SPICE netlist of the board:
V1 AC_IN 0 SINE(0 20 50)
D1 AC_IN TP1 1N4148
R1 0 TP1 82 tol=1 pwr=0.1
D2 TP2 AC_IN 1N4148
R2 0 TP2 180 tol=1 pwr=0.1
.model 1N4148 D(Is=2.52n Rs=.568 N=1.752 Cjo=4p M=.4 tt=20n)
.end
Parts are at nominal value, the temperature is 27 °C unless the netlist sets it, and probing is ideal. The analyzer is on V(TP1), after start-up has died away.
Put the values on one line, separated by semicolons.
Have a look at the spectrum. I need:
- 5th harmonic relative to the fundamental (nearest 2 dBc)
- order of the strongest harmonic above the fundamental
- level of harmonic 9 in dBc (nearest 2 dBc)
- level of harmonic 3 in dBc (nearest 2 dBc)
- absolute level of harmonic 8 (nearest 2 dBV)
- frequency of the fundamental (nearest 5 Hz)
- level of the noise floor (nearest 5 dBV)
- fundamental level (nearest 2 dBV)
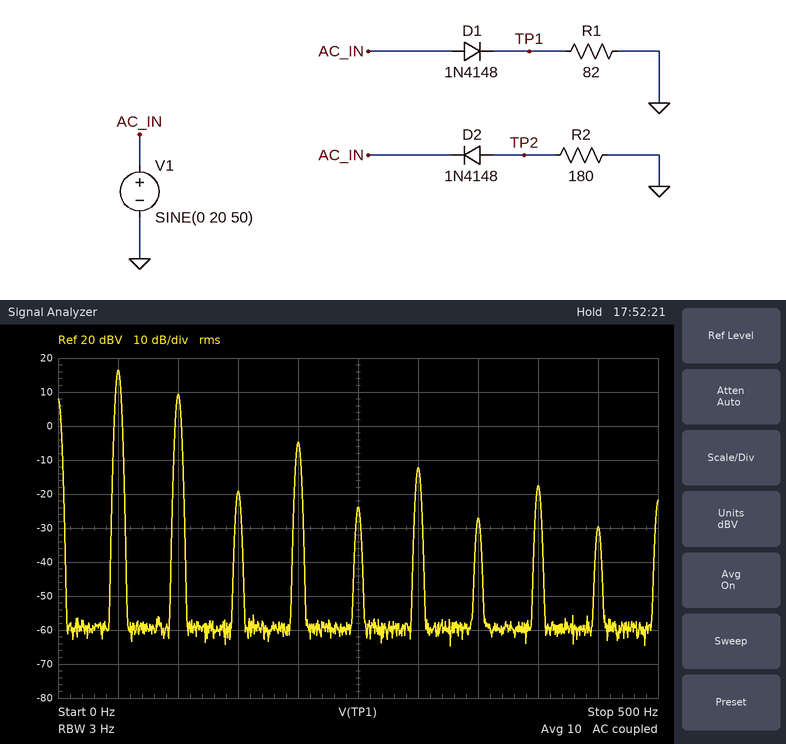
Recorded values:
-40 dBc; 2; -46 dBc; -36 dBc; -18 dBV; 50 Hz; -60 dBV; 16 dBV
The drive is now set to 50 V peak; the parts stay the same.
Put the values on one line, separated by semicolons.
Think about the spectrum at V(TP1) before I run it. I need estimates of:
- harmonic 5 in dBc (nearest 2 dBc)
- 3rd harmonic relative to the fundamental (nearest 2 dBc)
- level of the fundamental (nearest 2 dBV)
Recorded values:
-48 dBc; -44 dBc; 24 dBV
